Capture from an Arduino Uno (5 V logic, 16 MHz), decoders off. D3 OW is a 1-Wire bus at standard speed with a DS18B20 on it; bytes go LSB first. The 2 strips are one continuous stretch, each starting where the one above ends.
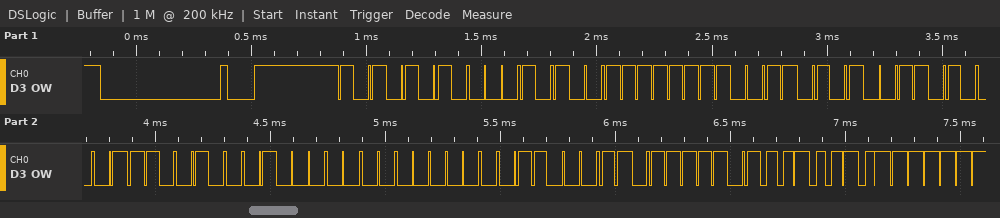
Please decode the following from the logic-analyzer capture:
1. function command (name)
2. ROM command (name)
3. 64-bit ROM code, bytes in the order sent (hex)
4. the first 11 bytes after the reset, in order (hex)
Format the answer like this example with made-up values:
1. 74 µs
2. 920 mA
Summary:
1. Read Scratchpad
2. Match ROM
3. 28 FF AC 2C 4E 04 00 C6
4. 55 28 FF AC 2C 4E 04 00 C6 BE A4
